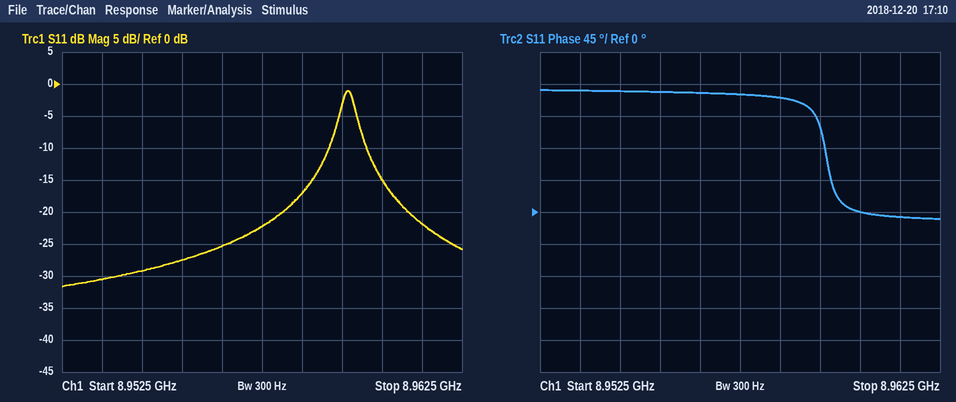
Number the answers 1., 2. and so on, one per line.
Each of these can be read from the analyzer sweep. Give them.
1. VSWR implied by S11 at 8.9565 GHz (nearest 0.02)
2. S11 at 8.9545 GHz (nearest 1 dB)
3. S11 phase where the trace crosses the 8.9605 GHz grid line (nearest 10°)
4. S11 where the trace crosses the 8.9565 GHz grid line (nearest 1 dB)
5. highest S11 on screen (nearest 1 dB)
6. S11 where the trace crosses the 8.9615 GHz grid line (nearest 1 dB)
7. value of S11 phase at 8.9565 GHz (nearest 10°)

1. 1.12
2. -29 dB
3. 0°
4. -25 dB
5. -1 dB
6. -22 dB
7. 170°
